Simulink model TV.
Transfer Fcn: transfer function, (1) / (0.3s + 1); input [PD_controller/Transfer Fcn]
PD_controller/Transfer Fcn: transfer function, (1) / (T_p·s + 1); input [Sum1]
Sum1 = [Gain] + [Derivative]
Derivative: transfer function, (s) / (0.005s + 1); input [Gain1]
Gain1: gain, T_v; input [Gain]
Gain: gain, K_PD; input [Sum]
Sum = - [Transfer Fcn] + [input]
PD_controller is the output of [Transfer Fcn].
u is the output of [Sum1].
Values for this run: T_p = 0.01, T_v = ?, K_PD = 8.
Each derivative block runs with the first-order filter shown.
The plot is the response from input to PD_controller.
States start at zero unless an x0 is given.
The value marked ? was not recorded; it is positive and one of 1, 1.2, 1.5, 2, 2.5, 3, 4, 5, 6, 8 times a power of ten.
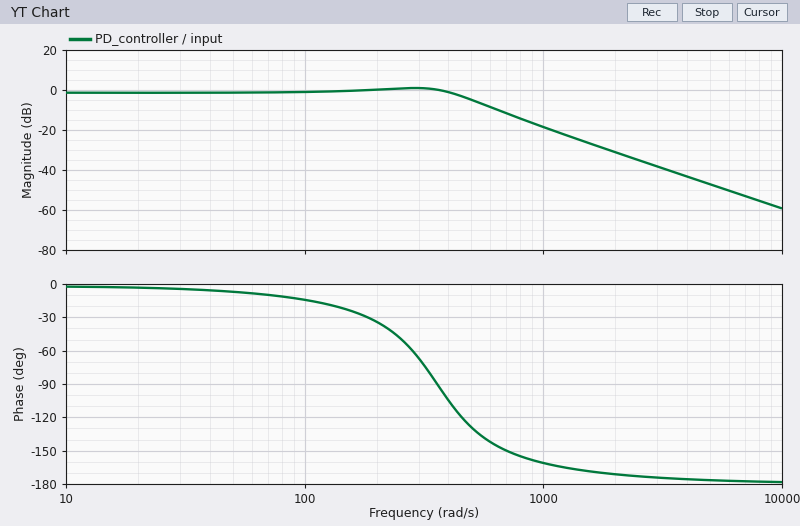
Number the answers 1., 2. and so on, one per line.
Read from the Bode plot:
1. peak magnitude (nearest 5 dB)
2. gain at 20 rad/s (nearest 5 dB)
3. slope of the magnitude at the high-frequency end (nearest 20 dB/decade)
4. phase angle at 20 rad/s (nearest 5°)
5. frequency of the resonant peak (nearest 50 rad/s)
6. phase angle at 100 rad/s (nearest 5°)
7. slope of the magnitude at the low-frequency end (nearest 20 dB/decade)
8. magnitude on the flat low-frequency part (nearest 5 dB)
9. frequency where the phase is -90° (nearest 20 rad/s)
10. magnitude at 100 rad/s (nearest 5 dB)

1. 0 dB
2. 0 dB
3. -40 dB/decade
4. -5°
5. 300 rad/s
6. -15°
7. 0 dB/decade
8. 0 dB
9. 360 rad/s
10. 0 dB
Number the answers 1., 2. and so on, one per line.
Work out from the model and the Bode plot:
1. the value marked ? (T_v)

1. 0.2
